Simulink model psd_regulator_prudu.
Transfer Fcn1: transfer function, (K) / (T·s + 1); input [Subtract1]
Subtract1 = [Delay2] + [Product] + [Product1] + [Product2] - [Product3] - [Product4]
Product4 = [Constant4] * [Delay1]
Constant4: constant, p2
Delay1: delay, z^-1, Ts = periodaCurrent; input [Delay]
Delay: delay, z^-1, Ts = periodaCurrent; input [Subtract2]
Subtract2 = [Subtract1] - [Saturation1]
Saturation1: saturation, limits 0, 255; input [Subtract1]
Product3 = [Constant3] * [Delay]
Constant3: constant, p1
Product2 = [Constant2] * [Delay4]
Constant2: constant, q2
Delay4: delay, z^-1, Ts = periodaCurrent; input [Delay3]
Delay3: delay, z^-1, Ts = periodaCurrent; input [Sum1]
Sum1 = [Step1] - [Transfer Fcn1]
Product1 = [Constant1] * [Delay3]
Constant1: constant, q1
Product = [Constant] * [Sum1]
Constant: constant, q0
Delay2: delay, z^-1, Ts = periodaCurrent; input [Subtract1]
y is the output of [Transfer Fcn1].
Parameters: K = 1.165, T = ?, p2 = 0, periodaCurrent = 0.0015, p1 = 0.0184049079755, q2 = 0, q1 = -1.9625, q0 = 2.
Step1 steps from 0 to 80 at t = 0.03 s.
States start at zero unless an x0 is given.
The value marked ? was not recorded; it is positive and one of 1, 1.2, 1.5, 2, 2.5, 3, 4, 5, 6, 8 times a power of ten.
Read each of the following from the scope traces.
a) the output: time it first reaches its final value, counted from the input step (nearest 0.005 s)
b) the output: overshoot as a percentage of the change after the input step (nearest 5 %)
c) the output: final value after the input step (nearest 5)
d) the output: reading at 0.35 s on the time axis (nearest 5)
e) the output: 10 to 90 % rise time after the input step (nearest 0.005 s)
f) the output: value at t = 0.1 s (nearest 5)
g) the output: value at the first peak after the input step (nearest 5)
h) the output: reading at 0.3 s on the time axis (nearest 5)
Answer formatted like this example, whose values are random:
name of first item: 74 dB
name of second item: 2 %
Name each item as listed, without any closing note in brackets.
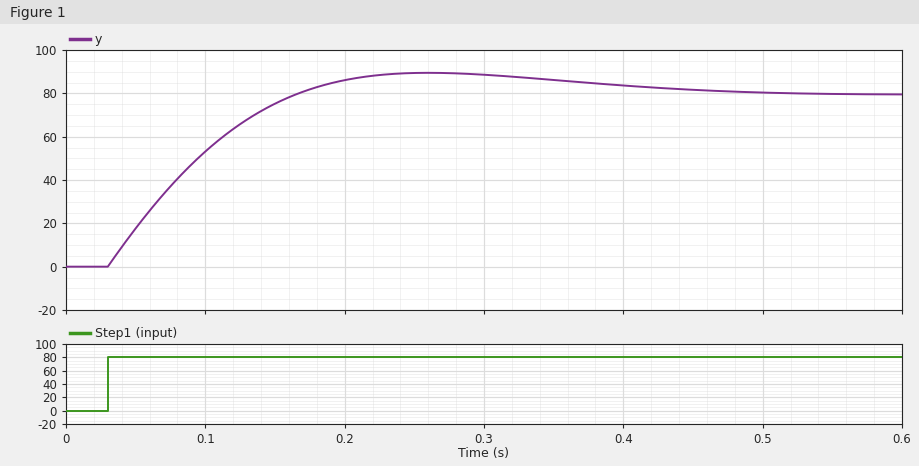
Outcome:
the output: time it first reaches its final value, counted from the input step: 0.135 s
the output: overshoot as a percentage of the change after the input step: 10 %
the output: final value after the input step: 80
the output: reading at 0.35 s on the time axis: 85
the output: 10 to 90 % rise time after the input step: 0.100 s
the output: value at t = 0.1 s: 55
the output: value at the first peak after the input step: 90
the output: reading at 0.3 s on the time axis: 90
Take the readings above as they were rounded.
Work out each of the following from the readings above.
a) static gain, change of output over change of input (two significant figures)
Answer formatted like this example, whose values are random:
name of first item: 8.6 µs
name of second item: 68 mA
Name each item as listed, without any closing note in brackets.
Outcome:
static gain, change of output over change of input: 1.0
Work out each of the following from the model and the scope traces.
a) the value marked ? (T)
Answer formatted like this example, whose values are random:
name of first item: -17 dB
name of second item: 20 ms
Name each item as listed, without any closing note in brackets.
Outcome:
the value marked ?: 0.2
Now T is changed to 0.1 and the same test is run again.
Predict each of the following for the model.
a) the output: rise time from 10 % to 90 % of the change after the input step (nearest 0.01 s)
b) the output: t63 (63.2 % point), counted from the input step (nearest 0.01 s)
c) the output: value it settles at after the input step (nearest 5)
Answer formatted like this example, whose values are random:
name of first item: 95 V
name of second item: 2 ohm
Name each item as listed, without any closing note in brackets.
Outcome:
the output: rise time from 10 % to 90 % of the change after the input step: 0.08 s
the output: t63 (63.2 % point), counted from the input step: 0.04 s
the output: value it settles at after the input step: 80
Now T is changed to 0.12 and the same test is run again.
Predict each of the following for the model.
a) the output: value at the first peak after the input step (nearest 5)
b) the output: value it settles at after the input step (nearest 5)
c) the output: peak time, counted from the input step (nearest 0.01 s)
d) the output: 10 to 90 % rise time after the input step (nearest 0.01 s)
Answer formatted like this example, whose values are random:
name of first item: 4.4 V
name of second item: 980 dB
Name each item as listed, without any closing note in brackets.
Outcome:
the output: value at the first peak after the input step: 85
the output: value it settles at after the input step: 80
the output: peak time, counted from the input step: 0.19 s
the output: 10 to 90 % rise time after the input step: 0.08 s
